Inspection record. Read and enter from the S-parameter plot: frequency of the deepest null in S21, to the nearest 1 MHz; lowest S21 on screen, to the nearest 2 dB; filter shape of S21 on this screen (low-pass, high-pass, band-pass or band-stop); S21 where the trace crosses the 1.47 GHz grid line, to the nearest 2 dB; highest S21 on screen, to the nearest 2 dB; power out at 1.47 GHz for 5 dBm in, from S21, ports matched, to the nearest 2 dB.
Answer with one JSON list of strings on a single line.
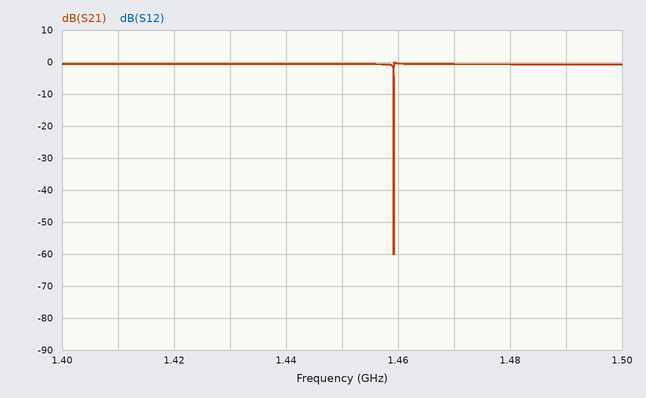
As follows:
["1.459 GHz", "-60 dB", "band-stop", "0 dB", "0 dB", "4 dBm"]
